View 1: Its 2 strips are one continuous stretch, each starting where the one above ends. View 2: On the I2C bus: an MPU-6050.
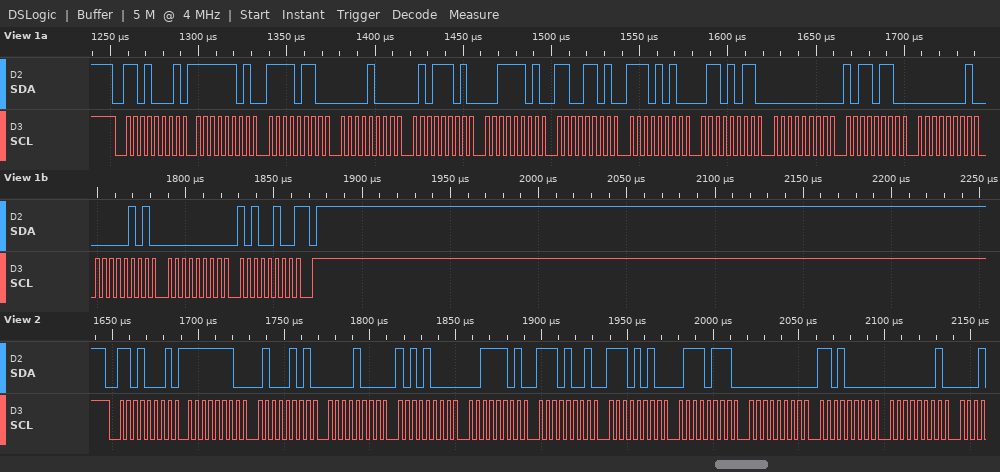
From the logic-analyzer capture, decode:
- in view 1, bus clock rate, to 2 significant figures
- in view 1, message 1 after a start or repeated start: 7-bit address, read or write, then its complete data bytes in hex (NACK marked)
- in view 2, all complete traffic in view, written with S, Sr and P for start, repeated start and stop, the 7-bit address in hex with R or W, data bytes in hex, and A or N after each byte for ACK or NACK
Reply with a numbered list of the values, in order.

1. 250 kHz
2. 0x68 read: FD F6 08 5D 3D CD EA 6B 00 B6 01 05 00 A4 NACK
3. S 68R A FE A 45 A 08 A A8 A 3D A E9 A EA A 77 A 00 A D0 A 01 A
